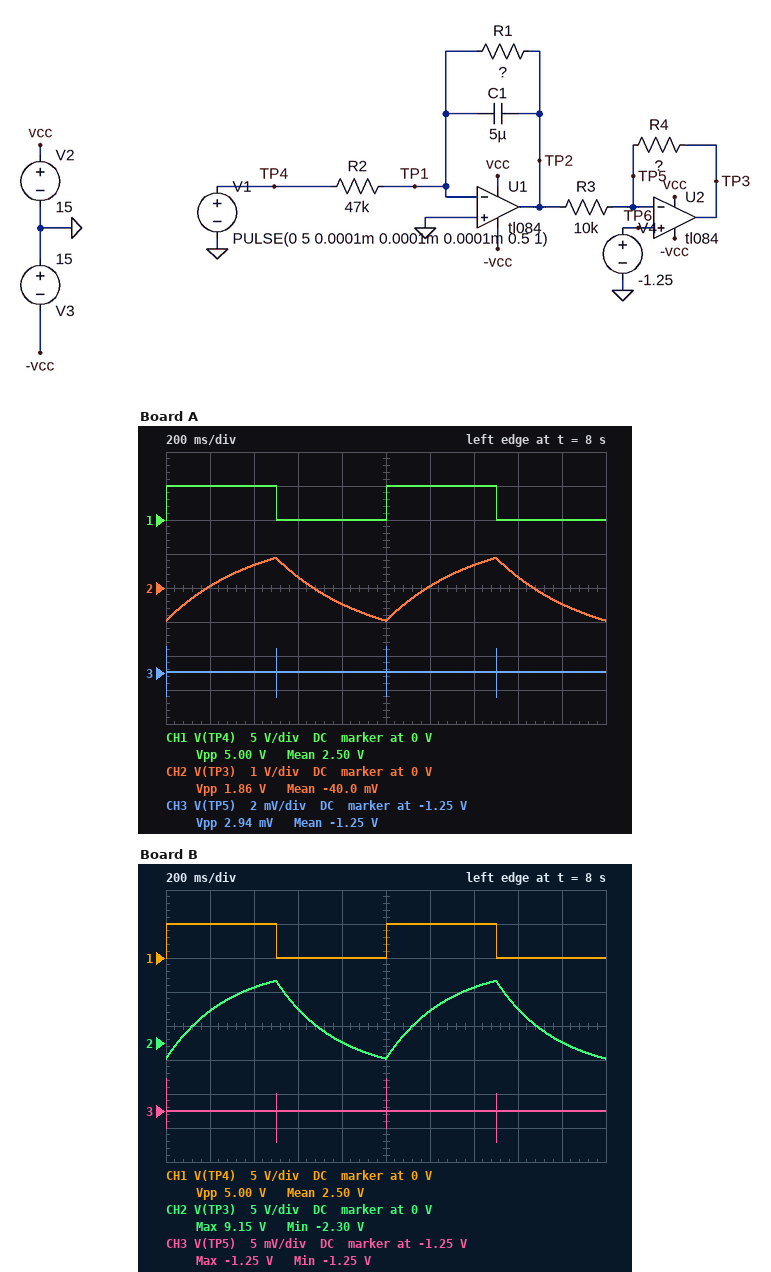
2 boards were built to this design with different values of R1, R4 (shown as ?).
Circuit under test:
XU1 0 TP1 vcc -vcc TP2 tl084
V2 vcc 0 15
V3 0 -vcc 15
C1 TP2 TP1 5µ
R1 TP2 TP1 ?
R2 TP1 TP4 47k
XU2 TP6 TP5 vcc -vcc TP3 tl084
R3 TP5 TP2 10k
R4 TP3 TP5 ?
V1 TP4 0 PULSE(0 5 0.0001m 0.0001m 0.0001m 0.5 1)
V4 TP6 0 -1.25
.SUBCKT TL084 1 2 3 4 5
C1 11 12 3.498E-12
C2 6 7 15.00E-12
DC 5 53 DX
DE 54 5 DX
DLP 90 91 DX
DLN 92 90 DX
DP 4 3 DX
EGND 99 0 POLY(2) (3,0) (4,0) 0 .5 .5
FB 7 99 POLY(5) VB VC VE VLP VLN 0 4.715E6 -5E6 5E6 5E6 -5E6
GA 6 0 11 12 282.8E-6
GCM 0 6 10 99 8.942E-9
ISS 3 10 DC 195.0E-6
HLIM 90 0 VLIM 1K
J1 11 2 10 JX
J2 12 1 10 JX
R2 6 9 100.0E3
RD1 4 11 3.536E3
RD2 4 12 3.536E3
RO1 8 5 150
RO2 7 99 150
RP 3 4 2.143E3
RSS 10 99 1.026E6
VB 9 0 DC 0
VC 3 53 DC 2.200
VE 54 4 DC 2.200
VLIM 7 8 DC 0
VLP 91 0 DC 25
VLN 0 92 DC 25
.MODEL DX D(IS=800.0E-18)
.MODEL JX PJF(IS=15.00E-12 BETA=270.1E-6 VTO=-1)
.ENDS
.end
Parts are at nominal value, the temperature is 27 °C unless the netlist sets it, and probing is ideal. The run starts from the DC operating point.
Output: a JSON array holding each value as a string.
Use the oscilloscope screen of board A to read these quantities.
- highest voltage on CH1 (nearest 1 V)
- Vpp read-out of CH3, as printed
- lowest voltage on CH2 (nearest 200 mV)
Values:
["5 V", "2.94 mV", "-1.0 V"]
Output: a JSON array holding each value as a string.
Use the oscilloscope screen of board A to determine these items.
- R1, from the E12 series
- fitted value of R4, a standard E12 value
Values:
["82 kΩ", "3.9 kΩ"]
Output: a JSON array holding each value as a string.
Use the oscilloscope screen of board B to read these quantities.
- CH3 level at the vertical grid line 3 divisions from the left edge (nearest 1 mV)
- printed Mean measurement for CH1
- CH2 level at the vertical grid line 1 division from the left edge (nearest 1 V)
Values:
["-1.250 V", "2.50 V", "5 V"]
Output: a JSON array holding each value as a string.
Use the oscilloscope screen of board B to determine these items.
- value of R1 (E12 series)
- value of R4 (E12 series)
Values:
["56 kΩ", "27 kΩ"]
